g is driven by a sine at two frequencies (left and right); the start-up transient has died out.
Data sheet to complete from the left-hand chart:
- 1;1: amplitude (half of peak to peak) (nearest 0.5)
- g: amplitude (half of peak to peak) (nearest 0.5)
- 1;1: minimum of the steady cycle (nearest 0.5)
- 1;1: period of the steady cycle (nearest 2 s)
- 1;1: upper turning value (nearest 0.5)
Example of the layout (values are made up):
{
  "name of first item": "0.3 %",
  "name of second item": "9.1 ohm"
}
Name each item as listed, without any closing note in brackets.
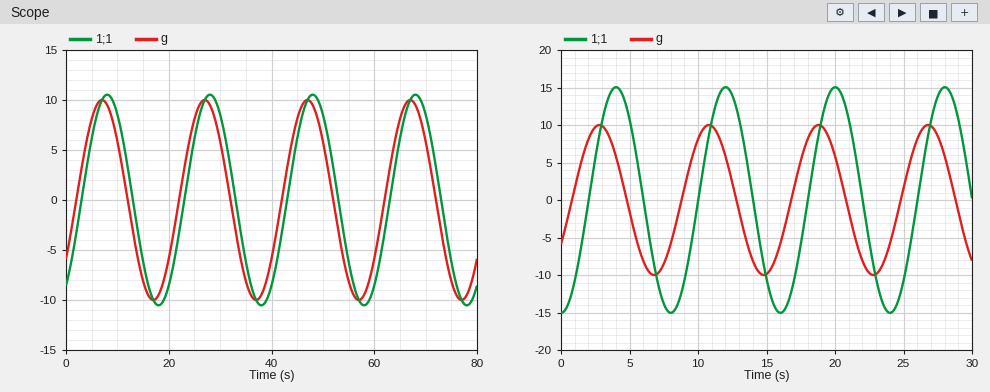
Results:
{
  "1;1: amplitude (half of peak to peak)": "10.5",
  "g: amplitude (half of peak to peak)": "10.0",
  "1;1: minimum of the steady cycle": "-10.5",
  "1;1: period of the steady cycle": "20 s",
  "1;1: upper turning value": "10.5"
}
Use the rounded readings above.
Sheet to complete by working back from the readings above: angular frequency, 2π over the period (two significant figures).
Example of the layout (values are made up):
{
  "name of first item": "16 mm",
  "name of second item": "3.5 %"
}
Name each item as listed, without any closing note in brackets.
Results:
{
  "angular frequency, 2π over the period": "0.31 rad/s"
}
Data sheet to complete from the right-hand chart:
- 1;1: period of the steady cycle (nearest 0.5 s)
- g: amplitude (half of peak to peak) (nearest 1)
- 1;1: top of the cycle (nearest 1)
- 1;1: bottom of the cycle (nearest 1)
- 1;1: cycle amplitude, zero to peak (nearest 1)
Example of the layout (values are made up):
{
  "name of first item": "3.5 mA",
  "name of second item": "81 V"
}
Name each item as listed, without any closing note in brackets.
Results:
{
  "1;1: period of the steady cycle": "8.0 s",
  "g: amplitude (half of peak to peak)": "10",
  "1;1: top of the cycle": "15",
  "1;1: bottom of the cycle": "-15",
  "1;1: cycle amplitude, zero to peak": "15"
}
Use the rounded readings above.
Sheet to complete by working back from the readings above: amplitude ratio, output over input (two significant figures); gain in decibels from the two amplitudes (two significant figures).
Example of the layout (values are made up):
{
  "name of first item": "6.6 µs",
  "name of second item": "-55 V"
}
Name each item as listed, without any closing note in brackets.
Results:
{
  "amplitude ratio, output over input": "1.5",
  "gain in decibels from the two amplitudes": "3.5 dB"
}
